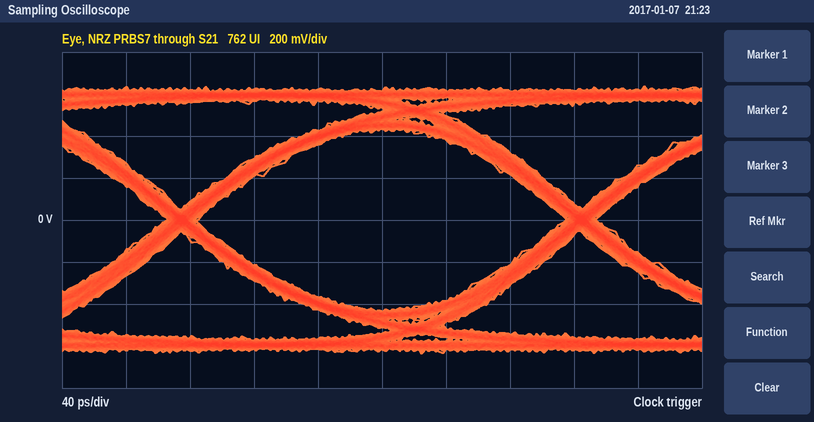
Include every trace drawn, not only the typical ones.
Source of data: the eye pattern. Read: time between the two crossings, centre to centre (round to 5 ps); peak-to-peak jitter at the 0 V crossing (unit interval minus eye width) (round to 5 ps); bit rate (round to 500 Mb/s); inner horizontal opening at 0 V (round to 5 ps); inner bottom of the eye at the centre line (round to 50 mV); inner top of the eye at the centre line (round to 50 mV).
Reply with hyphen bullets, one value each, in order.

- 250 ps
- 20 ps
- 4.0 Gb/s
- 230 ps
- -450 mV
- 450 mV
